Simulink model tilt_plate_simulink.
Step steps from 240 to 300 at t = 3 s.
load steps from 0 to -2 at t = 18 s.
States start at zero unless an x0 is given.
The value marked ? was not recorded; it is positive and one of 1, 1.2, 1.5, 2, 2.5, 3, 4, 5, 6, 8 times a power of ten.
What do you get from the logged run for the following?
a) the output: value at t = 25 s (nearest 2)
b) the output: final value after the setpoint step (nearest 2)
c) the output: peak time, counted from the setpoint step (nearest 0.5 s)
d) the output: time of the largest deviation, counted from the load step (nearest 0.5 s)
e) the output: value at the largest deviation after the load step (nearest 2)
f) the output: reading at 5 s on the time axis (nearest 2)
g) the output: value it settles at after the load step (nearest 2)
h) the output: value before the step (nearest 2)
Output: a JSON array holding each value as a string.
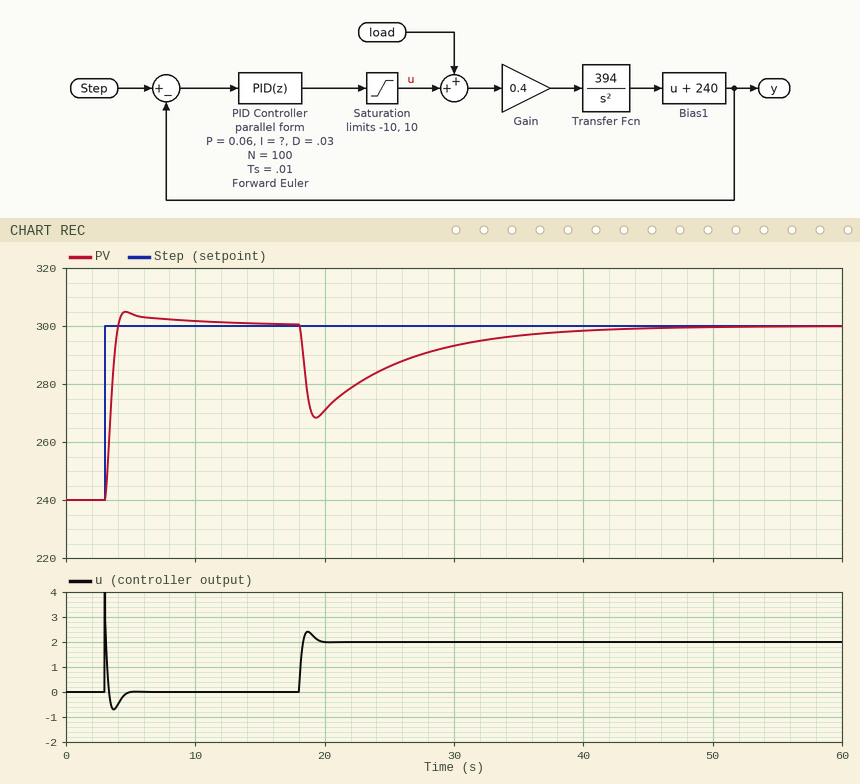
["286", "300", "1.5 s", "1.5 s", "268", "304", "300", "240"]
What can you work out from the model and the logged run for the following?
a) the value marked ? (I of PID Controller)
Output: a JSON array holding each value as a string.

["0.008"]
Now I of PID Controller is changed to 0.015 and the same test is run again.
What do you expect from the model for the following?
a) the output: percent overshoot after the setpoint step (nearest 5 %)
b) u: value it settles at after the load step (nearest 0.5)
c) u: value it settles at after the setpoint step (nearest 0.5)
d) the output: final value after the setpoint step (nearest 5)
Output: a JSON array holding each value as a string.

["15 %", "2.0", "0.0", "300"]
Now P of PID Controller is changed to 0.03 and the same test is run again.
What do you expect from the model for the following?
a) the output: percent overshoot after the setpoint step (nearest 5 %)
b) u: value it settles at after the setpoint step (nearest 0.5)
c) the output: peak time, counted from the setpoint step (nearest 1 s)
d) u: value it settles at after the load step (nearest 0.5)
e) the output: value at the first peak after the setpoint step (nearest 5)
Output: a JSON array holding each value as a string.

["15 %", "0.0", "3 s", "2.0", "310"]
